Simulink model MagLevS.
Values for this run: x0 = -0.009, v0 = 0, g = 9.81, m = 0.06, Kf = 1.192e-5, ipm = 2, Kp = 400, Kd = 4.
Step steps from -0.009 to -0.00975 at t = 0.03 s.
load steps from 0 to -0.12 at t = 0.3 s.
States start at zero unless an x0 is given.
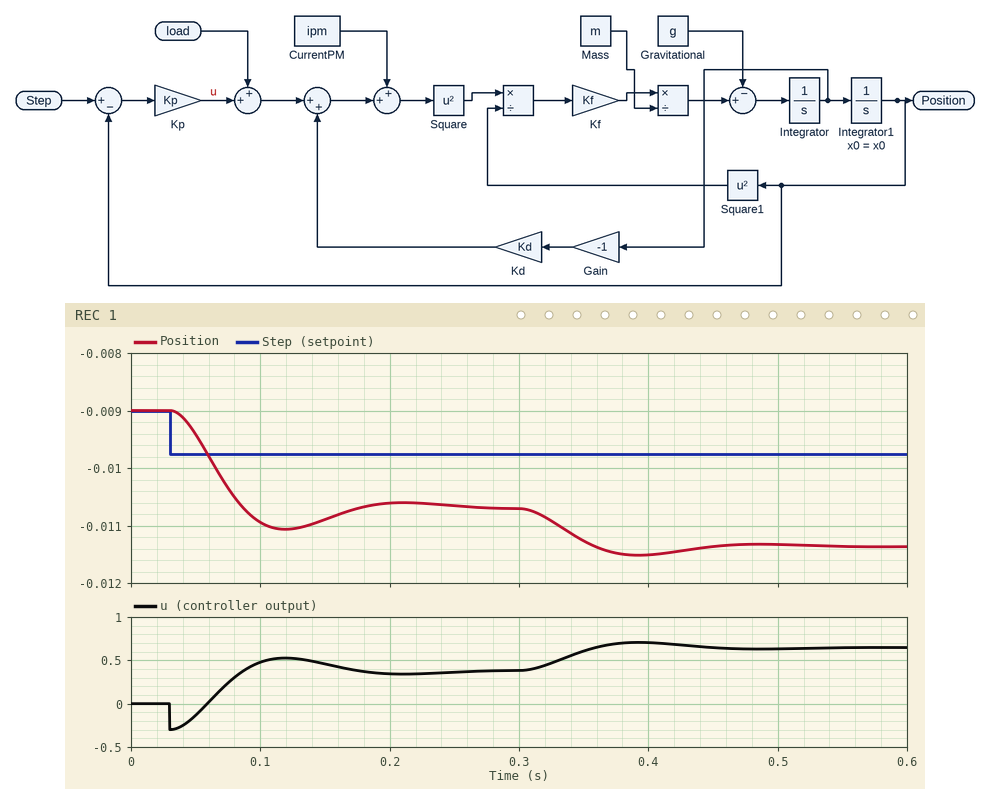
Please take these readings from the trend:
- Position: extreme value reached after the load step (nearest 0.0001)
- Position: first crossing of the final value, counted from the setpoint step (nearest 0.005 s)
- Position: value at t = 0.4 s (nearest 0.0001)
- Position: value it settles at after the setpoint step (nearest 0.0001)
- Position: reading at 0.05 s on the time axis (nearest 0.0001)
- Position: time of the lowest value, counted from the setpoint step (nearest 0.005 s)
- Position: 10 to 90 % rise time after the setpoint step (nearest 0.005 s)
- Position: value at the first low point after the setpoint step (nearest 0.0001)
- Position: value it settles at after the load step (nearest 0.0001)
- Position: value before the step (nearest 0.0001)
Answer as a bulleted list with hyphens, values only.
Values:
- -0.0115
- 0.055 s
- -0.0115
- -0.0107
- -0.0094
- 0.090 s
- 0.040 s
- -0.0111
- -0.0114
- -0.0090
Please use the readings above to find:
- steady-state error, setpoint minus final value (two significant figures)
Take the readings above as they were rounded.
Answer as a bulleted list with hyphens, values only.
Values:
- 0.00095
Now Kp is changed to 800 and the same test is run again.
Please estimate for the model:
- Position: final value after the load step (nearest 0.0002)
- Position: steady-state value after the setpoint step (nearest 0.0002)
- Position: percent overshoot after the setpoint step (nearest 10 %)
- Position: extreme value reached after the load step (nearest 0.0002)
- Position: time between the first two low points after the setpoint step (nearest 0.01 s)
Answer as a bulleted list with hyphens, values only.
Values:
- -0.0102
- -0.0100
- 40 %
- -0.0104
- 0.09 s
